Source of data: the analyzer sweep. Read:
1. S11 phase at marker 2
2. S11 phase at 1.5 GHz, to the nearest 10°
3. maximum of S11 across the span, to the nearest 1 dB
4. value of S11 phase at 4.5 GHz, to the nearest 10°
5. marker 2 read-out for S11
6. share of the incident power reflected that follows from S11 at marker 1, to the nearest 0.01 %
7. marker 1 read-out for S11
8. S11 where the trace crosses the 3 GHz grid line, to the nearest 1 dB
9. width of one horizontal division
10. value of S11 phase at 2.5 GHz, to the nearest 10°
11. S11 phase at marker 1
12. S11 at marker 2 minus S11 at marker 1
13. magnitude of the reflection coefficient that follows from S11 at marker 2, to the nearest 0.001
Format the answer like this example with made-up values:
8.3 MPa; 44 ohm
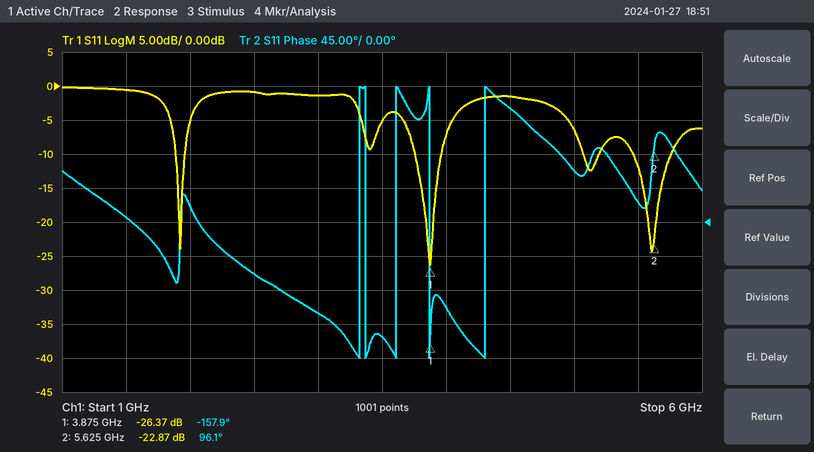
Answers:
96.1°; 10°; 0 dB; 150°; -22.87 dB; 0.23 %; -26.37 dB; -1 dB; 500 MHz; -70°; -157.9°; 3.50 dB; 0.072
